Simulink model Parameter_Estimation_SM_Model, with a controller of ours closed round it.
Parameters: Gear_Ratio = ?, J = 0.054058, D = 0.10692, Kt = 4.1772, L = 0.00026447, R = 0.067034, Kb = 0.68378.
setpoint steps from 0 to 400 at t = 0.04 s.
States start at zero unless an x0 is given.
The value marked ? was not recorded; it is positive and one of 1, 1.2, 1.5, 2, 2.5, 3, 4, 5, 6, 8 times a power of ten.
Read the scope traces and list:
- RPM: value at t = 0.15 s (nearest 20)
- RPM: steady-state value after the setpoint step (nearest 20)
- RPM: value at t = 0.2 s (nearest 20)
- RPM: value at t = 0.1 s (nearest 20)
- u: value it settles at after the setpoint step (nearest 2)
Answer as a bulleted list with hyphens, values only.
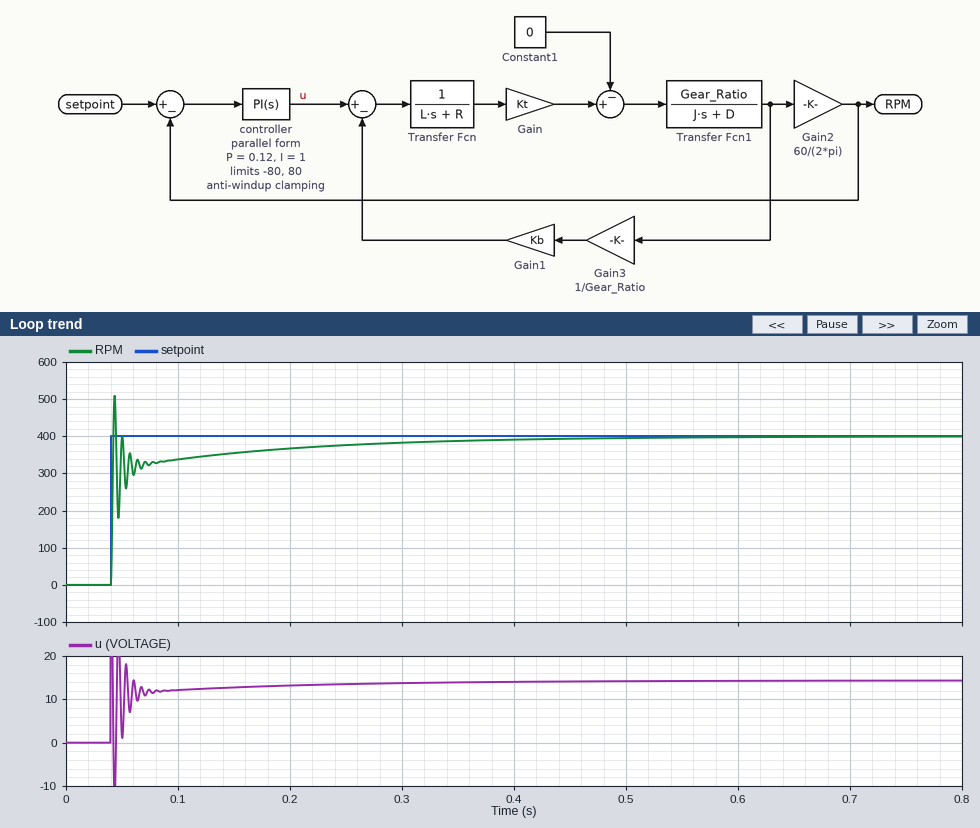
- 360
- 400
- 360
- 340
- 14
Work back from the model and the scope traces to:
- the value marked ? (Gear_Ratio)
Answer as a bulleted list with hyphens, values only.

- 2
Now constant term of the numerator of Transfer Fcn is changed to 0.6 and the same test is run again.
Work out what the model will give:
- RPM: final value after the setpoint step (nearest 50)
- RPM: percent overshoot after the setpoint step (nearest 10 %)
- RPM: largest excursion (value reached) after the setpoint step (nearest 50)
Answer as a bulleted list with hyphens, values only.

- 400
- 20 %
- 500
